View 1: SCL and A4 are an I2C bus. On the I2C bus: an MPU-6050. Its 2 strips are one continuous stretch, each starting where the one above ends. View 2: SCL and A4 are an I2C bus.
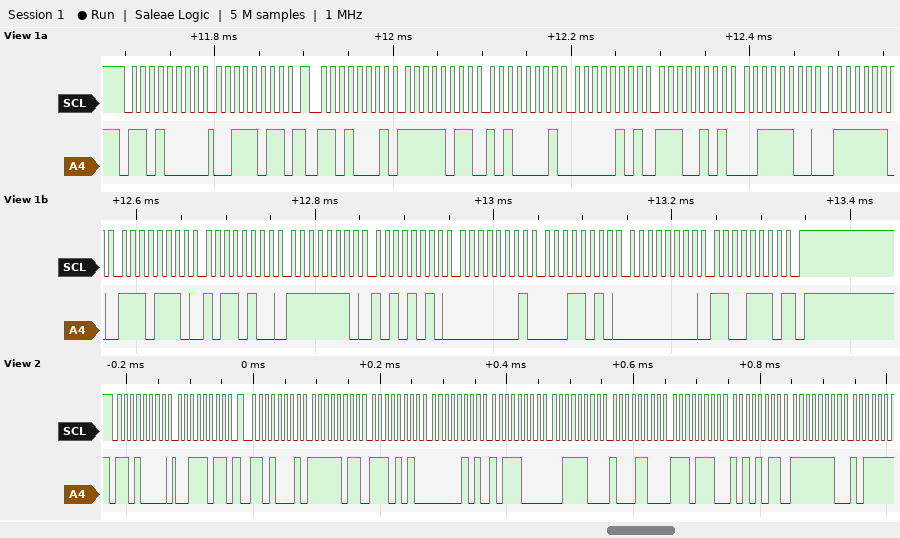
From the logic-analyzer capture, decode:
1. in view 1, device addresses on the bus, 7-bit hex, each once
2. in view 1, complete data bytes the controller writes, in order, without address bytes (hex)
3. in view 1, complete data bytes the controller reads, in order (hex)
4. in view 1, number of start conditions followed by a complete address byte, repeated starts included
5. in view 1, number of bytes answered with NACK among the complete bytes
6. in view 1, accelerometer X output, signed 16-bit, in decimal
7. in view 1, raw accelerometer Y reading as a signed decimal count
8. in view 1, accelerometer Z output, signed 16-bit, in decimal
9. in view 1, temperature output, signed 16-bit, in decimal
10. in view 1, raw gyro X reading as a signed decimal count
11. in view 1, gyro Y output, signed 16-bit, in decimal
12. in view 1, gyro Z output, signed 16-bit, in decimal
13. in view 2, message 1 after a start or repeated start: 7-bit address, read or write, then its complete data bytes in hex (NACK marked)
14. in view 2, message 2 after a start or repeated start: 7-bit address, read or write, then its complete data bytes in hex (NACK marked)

0x68
3B
FB A1 05 E5 3C 7E EE B4 FE AA 01 1A 00 CE
2
1
-1119
1509
15486
-4428
-342
282
206
0x68 write: 3B
0x68 read: FB EA 05 B8 3C 8C EE AB FE
